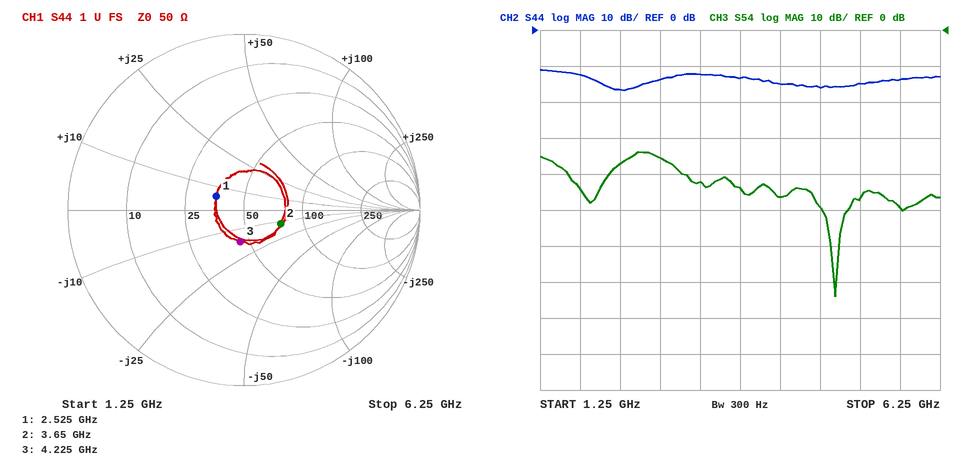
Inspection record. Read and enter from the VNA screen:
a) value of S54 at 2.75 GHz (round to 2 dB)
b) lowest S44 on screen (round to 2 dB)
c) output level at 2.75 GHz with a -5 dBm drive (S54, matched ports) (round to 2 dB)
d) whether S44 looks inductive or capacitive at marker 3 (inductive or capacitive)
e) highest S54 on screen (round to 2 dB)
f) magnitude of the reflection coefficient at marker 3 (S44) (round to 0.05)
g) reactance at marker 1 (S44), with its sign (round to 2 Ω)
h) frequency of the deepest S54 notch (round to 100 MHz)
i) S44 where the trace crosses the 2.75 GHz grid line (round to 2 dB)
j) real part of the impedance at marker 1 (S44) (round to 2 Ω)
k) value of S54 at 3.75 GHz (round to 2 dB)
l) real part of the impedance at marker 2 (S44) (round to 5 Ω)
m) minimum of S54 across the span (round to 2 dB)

-36 dB
-16 dB
-40 dBm
capacitive
-34 dB
0.20
+6 Ω
4.9 GHz
-14 dB
36 Ω
-44 dB
75 Ω
-74 dB
